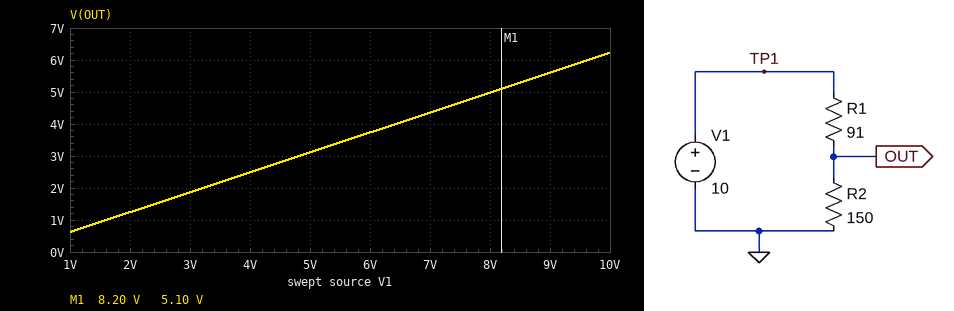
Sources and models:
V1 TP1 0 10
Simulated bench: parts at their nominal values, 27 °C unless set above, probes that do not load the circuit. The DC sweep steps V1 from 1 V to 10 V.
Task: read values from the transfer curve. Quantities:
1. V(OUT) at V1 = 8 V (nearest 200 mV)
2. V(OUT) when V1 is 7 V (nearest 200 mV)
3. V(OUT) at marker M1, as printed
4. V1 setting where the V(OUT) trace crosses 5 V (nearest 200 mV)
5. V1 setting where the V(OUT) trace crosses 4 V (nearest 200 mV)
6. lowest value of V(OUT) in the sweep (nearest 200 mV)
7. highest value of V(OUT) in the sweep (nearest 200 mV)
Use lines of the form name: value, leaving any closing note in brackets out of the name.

V(OUT) at V1 = 8 V: 5.0 V
V(OUT) when V1 is 7 V: 4.4 V
V(OUT) at marker M1, as printed: 5.10 V
V1 setting where the V(OUT) trace crosses 5 V: 8.0 V
V1 setting where the V(OUT) trace crosses 4 V: 6.4 V
lowest value of V(OUT) in the sweep: 600 mV
highest value of V(OUT) in the sweep: 6.2 V
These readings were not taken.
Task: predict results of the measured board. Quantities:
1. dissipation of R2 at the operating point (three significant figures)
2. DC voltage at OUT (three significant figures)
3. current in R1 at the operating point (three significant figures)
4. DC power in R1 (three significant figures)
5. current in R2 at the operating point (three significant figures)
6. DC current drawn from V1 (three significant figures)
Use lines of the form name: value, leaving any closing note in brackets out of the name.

dissipation of R2 at the operating point: 258 mW
DC voltage at OUT: 6.22 V
current in R1 at the operating point: 41.5 mA
DC power in R1: 157 mW
current in R2 at the operating point: 41.5 mA
DC current drawn from V1: 41.5 mA
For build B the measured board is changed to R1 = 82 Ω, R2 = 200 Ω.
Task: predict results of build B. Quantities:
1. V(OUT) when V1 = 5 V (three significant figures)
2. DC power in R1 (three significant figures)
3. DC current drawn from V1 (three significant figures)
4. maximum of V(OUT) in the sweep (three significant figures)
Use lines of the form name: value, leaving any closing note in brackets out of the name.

V(OUT) when V1 = 5 V: 3.55 V
DC power in R1: 103 mW
DC current drawn from V1: 35.5 mA
maximum of V(OUT) in the sweep: 7.09 V
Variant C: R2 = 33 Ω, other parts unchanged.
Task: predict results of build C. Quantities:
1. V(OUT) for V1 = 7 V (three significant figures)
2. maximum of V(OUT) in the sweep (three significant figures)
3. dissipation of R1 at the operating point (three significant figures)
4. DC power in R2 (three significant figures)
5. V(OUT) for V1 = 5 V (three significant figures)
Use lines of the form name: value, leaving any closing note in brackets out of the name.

V(OUT) for V1 = 7 V: 1.86 V
maximum of V(OUT) in the sweep: 2.66 V
dissipation of R1 at the operating point: 592 mW
DC power in R2: 215 mW
V(OUT) for V1 = 5 V: 1.33 V
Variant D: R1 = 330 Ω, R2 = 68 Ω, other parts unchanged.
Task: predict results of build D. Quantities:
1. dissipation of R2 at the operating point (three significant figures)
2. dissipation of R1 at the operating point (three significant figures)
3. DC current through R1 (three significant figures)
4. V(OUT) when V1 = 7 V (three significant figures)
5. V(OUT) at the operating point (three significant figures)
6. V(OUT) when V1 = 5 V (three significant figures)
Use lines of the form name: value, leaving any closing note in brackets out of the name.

dissipation of R2 at the operating point: 42.9 mW
dissipation of R1 at the operating point: 208 mW
DC current through R1: 25.1 mA
V(OUT) when V1 = 7 V: 1.20 V
V(OUT) at the operating point: 1.71 V
V(OUT) when V1 = 5 V: 854 mV
